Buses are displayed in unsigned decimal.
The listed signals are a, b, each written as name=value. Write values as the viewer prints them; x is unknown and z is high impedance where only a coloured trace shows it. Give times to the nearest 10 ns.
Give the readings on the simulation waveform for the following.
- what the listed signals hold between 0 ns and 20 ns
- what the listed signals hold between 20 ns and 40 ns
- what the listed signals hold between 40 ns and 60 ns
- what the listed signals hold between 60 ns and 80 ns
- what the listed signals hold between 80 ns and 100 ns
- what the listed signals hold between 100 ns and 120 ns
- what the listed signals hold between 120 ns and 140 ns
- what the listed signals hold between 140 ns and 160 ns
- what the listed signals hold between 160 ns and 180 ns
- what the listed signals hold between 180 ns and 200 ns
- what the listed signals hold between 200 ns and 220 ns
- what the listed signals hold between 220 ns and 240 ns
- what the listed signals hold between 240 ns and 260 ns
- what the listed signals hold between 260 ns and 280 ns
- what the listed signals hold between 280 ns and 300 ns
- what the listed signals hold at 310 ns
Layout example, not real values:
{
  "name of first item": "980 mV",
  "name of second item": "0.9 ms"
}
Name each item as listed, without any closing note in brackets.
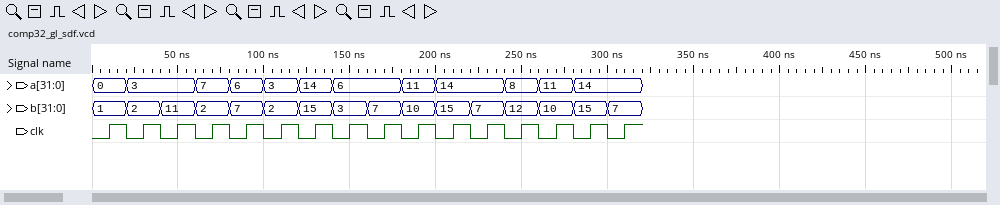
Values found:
{
  "what the listed signals hold between 0 ns and 20 ns": "a=0, b=1",
  "what the listed signals hold between 20 ns and 40 ns": "a=3, b=2",
  "what the listed signals hold between 40 ns and 60 ns": "a=3, b=11",
  "what the listed signals hold between 60 ns and 80 ns": "a=7, b=2",
  "what the listed signals hold between 80 ns and 100 ns": "a=6, b=7",
  "what the listed signals hold between 100 ns and 120 ns": "a=3, b=2",
  "what the listed signals hold between 120 ns and 140 ns": "a=14, b=15",
  "what the listed signals hold between 140 ns and 160 ns": "a=6, b=3",
  "what the listed signals hold between 160 ns and 180 ns": "a=6, b=7",
  "what the listed signals hold between 180 ns and 200 ns": "a=11, b=10",
  "what the listed signals hold between 200 ns and 220 ns": "a=14, b=15",
  "what the listed signals hold between 220 ns and 240 ns": "a=14, b=7",
  "what the listed signals hold between 240 ns and 260 ns": "a=8, b=12",
  "what the listed signals hold between 260 ns and 280 ns": "a=11, b=10",
  "what the listed signals hold between 280 ns and 300 ns": "a=14, b=15",
  "what the listed signals hold at 310 ns": "a=14, b=7"
}
